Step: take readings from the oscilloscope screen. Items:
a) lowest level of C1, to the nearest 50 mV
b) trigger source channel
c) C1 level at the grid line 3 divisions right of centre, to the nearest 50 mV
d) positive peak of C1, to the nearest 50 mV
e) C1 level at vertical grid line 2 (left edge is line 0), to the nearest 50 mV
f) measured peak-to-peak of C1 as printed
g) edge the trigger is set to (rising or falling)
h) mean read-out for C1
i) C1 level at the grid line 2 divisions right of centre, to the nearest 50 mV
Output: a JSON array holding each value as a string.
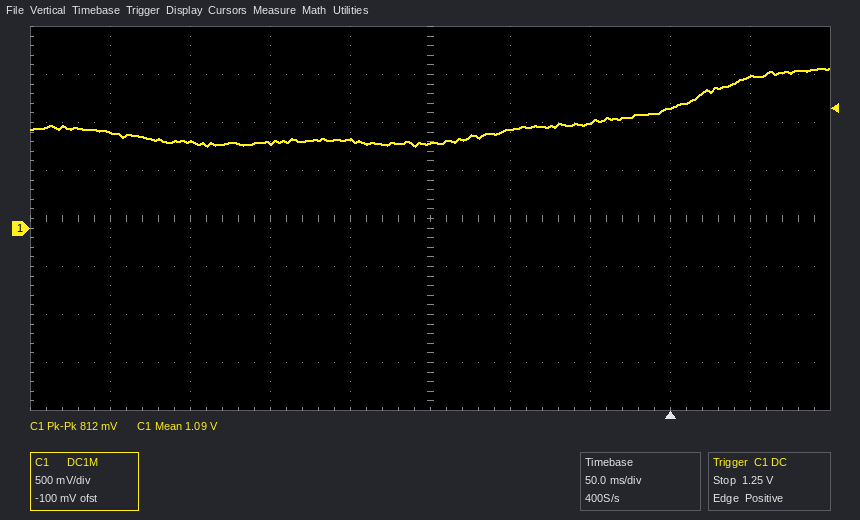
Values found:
["850 mV", "C1", "1.25 V", "1.65 V", "900 mV", "812 mV", "rising", "1.09 V", "1.10 V"]
